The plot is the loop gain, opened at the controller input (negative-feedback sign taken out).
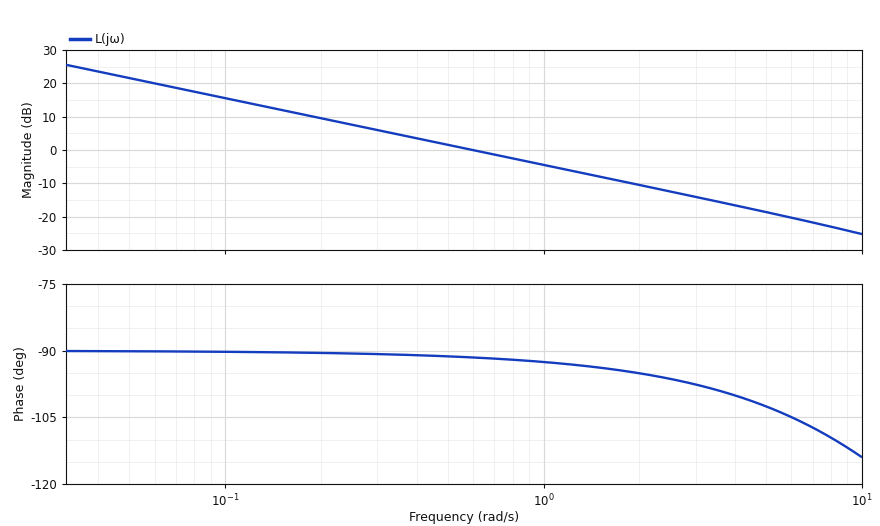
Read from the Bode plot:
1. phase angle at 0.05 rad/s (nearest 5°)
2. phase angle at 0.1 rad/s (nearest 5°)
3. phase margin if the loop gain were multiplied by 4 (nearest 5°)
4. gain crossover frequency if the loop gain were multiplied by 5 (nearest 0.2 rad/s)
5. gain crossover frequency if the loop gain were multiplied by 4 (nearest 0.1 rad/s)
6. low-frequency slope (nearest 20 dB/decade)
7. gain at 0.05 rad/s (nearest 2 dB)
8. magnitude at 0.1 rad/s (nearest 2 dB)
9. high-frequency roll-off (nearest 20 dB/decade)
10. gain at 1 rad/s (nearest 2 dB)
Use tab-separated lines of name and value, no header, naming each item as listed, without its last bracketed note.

phase angle at 0.05 rad/s	-90°
phase angle at 0.1 rad/s	-90°
phase margin if the loop gain were multiplied by 4	85°
gain crossover frequency if the loop gain were multiplied by 5	3.0 rad/s
gain crossover frequency if the loop gain were multiplied by 4	2.4 rad/s
low-frequency slope	-20 dB/decade
gain at 0.05 rad/s	22 dB
magnitude at 0.1 rad/s	16 dB
high-frequency roll-off	-20 dB/decade
gain at 1 rad/s	-4 dB
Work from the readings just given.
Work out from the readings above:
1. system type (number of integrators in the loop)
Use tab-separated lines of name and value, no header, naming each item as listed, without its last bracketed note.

system type	1
